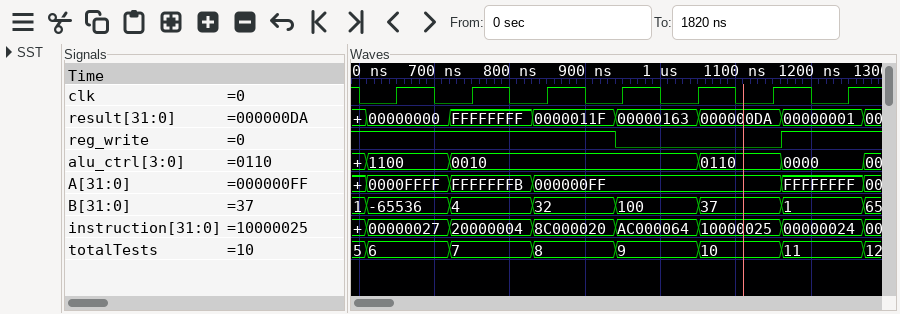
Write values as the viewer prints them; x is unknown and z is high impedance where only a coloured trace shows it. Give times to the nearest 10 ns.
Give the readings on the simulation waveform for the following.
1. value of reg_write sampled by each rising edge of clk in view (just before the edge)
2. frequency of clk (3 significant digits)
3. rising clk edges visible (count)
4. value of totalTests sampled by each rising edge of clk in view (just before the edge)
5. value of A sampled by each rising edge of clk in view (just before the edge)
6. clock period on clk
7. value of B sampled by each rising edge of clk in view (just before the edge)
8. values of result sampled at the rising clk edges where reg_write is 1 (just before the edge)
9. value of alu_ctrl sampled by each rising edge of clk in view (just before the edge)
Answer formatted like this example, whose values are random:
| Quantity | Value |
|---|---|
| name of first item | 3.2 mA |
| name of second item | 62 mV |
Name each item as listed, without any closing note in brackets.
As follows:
| Quantity | Value |
|---|---|
| value of reg_write sampled by each rising edge of clk in view | 1 1 1 0 0 0 1 |
| frequency of clk | 10.0 MHz |
| rising clk edges visible | 7 |
| value of totalTests sampled by each rising edge of clk in view | 6, 7, 8, 9, 9, 10, 11 |
| value of A sampled by each rising edge of clk in view | 0000FFFF, FFFFFFFB, 000000FF, 000000FF, 000000FF, 000000FF, FFFFFFFF |
| clock period on clk | 100 ns |
| value of B sampled by each rising edge of clk in view | -65536, 4, 32, 100, 100, 37, 1 |
| values of result sampled at the rising clk edges where reg_write is 1 | 00000000, FFFFFFFF, 0000011F, 00000001 |
| value of alu_ctrl sampled by each rising edge of clk in view | 1100, 0010, 0010, 0010, 0010, 0110, 0000 |
